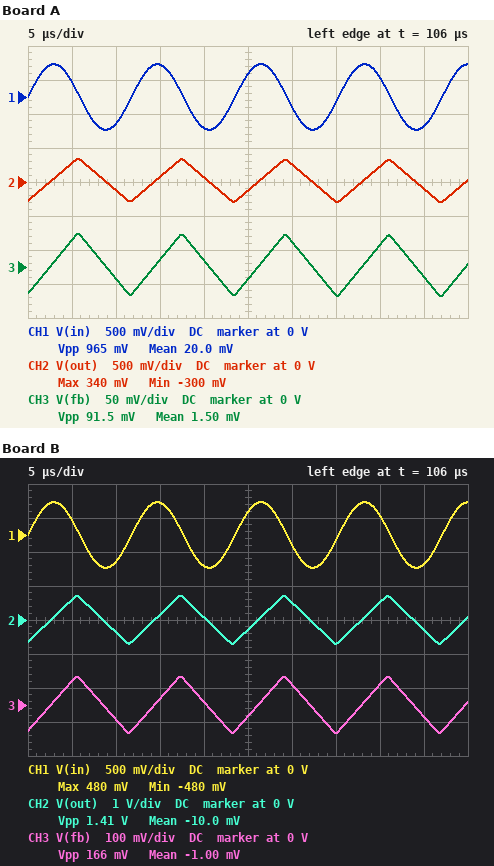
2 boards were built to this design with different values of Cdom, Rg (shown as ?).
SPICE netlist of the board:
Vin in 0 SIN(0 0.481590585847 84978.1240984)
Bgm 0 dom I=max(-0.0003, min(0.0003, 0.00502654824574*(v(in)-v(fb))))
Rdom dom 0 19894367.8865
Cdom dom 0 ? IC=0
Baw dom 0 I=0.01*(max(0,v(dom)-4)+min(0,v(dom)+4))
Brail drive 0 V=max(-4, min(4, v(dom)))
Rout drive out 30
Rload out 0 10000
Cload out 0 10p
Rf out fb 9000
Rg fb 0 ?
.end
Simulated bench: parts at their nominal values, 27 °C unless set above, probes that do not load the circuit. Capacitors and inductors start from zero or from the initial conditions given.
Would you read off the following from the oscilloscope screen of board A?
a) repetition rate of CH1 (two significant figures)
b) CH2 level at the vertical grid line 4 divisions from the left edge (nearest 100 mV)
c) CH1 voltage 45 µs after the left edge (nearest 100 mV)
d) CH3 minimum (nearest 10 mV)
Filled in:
85 kHz
100 mV
-400 mV
-40 mV
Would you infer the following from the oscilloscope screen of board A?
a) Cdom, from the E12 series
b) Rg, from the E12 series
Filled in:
2.7 nF
1.5 kΩ
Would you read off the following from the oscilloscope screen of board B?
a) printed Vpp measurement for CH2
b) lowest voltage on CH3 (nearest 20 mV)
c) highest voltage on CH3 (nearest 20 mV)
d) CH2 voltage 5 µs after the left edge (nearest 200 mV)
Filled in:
1.41 V
-80 mV
80 mV
600 mV
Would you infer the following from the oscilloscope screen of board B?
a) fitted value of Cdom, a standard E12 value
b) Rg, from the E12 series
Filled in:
1.2 nF
1.2 kΩ
